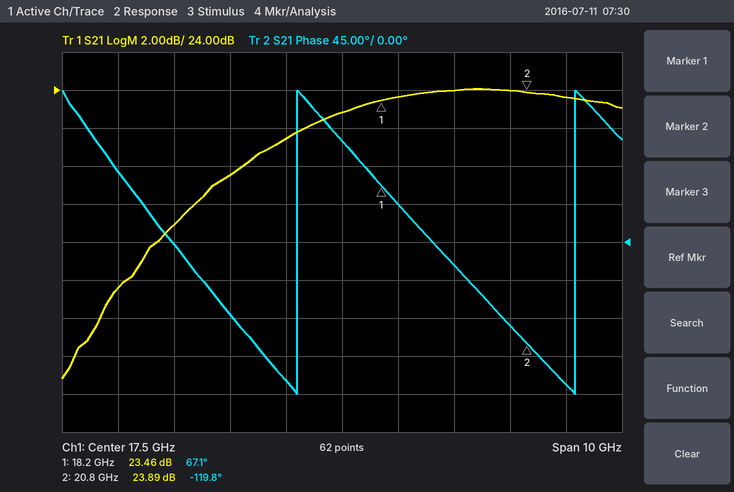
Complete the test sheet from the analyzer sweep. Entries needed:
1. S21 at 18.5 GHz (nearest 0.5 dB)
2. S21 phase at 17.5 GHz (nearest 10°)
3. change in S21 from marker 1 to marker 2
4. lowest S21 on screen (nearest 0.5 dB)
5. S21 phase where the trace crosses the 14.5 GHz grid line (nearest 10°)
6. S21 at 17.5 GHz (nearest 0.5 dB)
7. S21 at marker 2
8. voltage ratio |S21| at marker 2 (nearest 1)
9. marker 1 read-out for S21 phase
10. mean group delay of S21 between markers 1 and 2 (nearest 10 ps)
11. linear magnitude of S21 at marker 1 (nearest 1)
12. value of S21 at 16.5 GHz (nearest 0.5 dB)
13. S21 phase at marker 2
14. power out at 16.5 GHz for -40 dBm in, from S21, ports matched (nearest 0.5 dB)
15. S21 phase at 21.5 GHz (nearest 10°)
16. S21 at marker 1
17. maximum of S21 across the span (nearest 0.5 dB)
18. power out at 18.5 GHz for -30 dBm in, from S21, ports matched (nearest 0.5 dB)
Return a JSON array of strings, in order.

["23.5 dB", "120°", "0.43 dB", "9.0 dB", "0°", "23.0 dB", "23.89 dB", "16", "67.1°", "200 ps", "15", "21.5 dB", "-119.8°", "-18.5 dBm", "-170°", "23.46 dB", "24.0 dB", "-6.5 dBm"]
